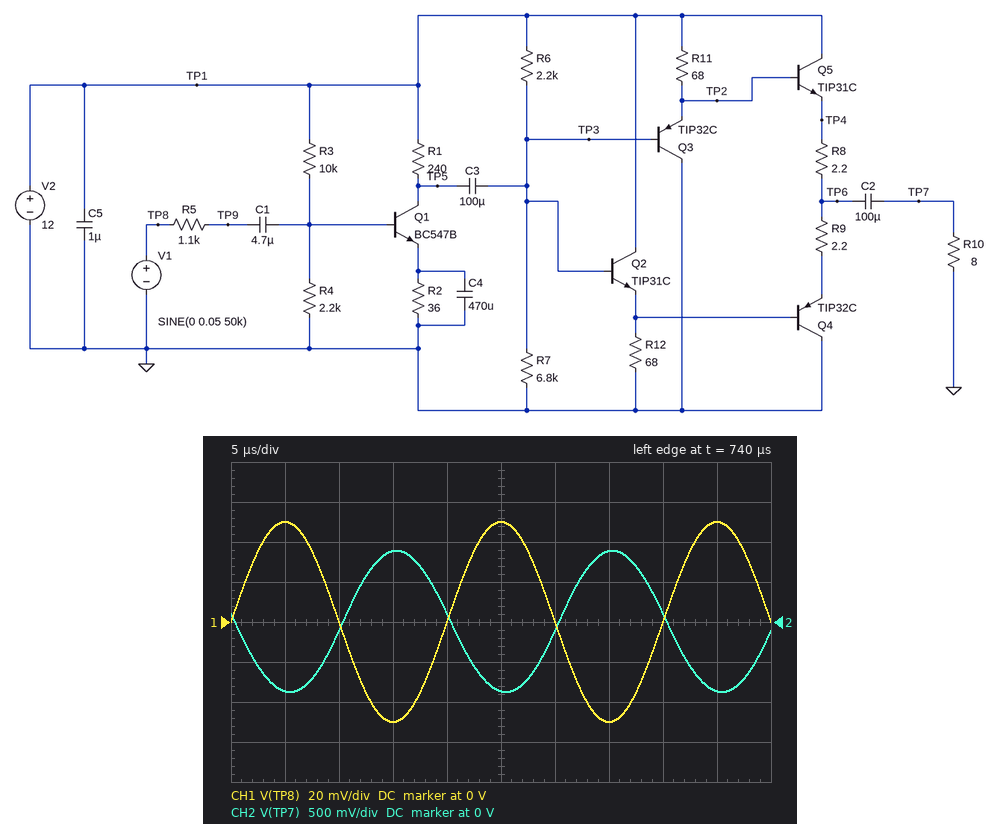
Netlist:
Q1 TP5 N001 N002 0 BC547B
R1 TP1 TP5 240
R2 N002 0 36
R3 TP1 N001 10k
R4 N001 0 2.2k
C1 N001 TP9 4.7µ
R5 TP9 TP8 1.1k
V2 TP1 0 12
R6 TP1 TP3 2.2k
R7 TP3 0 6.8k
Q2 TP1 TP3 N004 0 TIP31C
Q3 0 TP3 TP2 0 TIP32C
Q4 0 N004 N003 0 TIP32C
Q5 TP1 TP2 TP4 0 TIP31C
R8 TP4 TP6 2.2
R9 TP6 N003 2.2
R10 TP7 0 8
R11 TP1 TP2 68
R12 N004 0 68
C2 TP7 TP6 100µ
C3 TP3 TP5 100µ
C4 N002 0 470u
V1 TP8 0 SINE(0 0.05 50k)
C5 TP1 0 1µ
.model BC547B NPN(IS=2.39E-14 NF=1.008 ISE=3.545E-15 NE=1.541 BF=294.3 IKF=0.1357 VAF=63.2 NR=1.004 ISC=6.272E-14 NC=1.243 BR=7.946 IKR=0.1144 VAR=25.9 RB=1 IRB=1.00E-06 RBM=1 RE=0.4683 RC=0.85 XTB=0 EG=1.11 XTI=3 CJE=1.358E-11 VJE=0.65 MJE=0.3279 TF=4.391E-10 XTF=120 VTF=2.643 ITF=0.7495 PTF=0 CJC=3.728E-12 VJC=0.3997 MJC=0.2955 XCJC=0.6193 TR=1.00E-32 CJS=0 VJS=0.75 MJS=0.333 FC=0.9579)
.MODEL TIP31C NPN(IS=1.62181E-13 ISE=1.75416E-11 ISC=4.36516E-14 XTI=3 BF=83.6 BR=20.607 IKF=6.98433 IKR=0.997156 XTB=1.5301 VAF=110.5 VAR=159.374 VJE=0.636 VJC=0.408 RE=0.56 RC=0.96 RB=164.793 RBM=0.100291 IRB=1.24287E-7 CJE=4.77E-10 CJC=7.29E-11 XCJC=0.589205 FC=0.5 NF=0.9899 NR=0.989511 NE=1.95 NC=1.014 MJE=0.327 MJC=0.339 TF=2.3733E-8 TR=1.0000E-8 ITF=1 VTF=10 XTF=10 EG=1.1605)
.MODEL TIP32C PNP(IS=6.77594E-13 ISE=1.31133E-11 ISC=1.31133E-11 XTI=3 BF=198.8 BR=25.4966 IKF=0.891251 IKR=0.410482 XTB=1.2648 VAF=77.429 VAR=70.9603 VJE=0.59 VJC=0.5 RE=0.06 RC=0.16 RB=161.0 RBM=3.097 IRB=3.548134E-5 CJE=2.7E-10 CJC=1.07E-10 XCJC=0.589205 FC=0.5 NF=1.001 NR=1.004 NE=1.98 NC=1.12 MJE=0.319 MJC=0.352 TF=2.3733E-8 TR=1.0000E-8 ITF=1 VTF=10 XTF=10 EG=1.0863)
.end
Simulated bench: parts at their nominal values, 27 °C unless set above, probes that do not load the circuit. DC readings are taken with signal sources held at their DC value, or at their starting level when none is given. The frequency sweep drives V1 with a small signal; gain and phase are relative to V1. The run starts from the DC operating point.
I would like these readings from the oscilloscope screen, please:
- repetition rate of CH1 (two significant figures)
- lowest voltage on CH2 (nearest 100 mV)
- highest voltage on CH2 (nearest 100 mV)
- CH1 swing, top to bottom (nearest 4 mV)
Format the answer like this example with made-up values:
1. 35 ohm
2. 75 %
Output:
1. 50 kHz
2. -900 mV
3. 900 mV
4. 100 mV
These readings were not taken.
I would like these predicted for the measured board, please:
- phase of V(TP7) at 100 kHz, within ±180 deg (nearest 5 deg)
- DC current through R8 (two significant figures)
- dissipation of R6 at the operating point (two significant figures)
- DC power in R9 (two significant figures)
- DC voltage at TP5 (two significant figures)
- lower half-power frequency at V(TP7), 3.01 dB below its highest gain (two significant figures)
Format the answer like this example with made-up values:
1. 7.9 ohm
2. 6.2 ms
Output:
1. 165 deg
2. 24 mA
3. 8.9 mW
4. 1.3 mW
5. 4.2 V
6. 200 Hz
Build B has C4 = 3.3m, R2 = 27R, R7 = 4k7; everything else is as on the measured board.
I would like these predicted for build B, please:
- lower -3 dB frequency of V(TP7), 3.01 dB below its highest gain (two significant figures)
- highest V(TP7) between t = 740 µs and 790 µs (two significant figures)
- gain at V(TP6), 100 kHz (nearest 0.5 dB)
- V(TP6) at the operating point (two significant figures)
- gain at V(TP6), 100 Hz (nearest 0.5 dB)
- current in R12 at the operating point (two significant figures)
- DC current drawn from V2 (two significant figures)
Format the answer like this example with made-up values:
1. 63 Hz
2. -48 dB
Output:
1. 170 Hz
2. 830 mV
3. 24.5 dB
4. 7.0 V
5. 25.5 dB
6. 92 mA
7. 220 mA
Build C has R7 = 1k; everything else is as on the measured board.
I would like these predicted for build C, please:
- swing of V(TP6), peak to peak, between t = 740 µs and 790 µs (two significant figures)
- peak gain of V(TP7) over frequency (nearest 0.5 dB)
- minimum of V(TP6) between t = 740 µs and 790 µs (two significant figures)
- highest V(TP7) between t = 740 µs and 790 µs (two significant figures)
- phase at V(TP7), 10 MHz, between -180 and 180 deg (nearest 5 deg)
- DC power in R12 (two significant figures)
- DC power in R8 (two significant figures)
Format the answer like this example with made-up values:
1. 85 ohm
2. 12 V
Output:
1. 1.5 V
2. 24.0 dB
3. 3.0 V
4. 770 mV
5. 40 deg
6. 140 mW
7. 1.0 mW
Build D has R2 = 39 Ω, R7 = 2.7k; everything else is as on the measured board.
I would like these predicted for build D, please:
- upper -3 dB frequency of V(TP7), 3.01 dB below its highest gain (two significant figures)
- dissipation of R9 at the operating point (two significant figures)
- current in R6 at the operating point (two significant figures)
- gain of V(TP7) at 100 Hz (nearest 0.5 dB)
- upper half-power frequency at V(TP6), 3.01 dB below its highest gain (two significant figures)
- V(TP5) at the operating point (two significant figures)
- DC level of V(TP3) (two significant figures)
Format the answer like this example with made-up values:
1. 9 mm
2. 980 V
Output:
1. 580 kHz
2. 1.2 mW
3. 2.7 mA
4. 17.0 dB
5. 570 kHz
6. 4.7 V
7. 6.0 V
